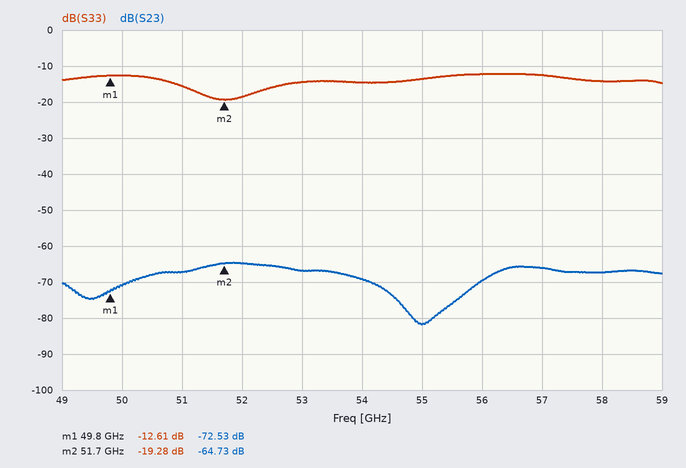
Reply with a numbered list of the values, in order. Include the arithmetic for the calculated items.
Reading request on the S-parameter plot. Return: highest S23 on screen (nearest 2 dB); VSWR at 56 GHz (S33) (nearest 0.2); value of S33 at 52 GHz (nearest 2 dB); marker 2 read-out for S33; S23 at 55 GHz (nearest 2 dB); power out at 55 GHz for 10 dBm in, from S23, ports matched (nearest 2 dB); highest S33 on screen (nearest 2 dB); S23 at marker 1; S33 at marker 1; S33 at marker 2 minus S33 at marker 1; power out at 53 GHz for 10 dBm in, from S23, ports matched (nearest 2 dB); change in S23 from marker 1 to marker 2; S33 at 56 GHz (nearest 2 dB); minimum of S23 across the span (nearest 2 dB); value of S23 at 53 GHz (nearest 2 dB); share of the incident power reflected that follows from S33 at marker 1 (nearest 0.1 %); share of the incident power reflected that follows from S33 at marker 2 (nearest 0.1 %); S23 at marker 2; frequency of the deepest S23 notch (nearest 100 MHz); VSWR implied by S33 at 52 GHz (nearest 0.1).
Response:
1. -64 dB
2. |Γ| = 10^(-12/20) = 0.2512; VSWR = (1 + 0.2512)/(1 − 0.2512) ≈ 1.67, so 1.6 to the nearest 0.2
3. -18 dB
4. -19.28 dB
5. -82 dB
6. 10 dBm + (-82 dB) = -72 dBm
7. -12 dB
8. -72.53 dB
9. -12.61 dB
10. -19.28 − (-12.61) = -6.67 dB
11. 10 dBm + (-66 dB) = -56 dBm
12. -64.73 − (-72.53) = 7.80 dB
13. -12 dB
14. -82 dB
15. -66 dB
16. 10^(-12.61/10) ≈ 5.5 %
17. 10^(-19.28/10) ≈ 1.2 %
18. -64.73 dB
19. 55.0 GHz
20. |Γ| = 10^(-18/20) = 0.1259; VSWR = (1 + 0.1259)/(1 − 0.1259) ≈ 1.3
